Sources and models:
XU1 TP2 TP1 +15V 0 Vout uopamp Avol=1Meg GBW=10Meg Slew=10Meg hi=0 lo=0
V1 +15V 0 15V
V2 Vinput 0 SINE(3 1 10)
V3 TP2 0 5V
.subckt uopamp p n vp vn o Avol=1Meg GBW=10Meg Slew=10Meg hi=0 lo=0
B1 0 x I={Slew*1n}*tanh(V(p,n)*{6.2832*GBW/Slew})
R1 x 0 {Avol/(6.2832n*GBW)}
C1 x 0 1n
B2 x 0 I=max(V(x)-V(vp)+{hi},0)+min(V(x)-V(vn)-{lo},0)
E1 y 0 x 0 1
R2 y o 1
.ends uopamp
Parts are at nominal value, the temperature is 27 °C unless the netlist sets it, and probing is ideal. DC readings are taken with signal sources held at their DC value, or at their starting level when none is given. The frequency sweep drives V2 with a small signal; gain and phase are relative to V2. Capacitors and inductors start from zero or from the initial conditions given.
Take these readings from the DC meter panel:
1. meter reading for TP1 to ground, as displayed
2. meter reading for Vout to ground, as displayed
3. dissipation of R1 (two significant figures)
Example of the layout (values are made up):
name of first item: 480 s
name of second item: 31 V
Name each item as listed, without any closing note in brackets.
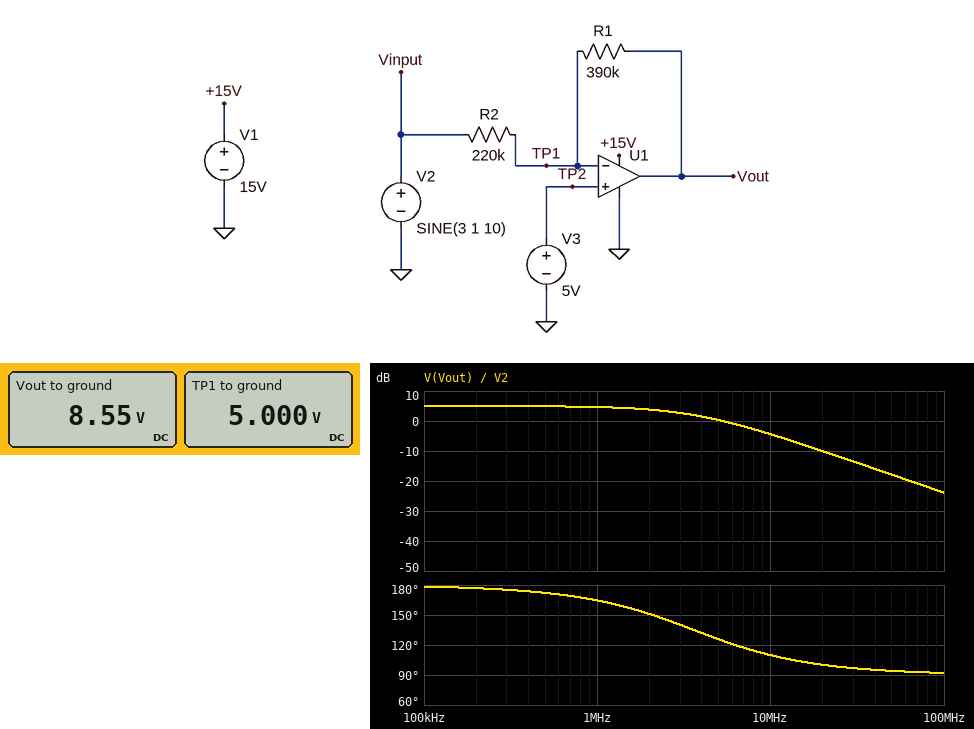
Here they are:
meter reading for TP1 to ground, as displayed: 5.000 V
meter reading for Vout to ground, as displayed: 8.55 V
dissipation of R1: 32 µW
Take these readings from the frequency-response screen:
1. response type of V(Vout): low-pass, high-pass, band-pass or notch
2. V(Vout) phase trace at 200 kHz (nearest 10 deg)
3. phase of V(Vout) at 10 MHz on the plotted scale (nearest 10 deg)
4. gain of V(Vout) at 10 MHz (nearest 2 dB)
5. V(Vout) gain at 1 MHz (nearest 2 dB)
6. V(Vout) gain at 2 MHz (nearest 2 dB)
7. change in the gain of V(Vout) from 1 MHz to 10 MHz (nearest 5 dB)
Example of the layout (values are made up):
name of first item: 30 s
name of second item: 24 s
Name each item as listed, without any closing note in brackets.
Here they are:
response type of V(Vout): low-pass, high-pass, band-pass or notch: low-pass
V(Vout) phase trace at 200 kHz: 180 deg
phase of V(Vout) at 10 MHz on the plotted scale: 110 deg
gain of V(Vout) at 10 MHz: -4 dB
V(Vout) gain at 1 MHz: 4 dB
V(Vout) gain at 2 MHz: 4 dB
change in the gain of V(Vout) from 1 MHz to 10 MHz: -10 dB
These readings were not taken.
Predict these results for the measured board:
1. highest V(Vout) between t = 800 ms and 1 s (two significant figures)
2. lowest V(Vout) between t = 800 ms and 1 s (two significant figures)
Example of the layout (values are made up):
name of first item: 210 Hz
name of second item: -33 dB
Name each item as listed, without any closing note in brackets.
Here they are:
highest V(Vout) between t = 800 ms and 1 s: 10 V
lowest V(Vout) between t = 800 ms and 1 s: 6.8 V
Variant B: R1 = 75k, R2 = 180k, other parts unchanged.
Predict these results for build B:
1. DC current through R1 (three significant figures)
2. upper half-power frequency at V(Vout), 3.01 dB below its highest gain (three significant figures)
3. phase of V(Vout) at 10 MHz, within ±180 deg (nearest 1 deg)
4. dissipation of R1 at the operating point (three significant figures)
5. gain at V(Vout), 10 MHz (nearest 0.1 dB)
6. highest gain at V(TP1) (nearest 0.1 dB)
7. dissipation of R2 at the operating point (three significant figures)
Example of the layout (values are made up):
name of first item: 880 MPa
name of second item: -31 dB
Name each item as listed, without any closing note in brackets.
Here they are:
DC current through R1: 11.1 µA
upper half-power frequency at V(Vout), 3.01 dB below its highest gain: 7.06 MHz
phase of V(Vout) at 10 MHz, within ±180 deg: 125 deg
dissipation of R1 at the operating point: 9.26 µW
gain at V(Vout), 10 MHz: -12.4 dB
highest gain at V(TP1): -10.6 dB
dissipation of R2 at the operating point: 22.2 µW
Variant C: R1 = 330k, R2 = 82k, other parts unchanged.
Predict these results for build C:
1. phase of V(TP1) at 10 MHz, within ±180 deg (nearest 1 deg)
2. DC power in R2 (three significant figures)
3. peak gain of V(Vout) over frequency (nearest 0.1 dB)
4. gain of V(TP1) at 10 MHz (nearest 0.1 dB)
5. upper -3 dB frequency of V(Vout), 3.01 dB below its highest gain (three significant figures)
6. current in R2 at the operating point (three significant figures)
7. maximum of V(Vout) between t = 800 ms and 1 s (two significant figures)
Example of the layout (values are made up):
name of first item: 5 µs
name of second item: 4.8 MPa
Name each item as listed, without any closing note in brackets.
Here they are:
phase of V(TP1) at 10 MHz, within ±180 deg: 11 deg
DC power in R2: 48.8 µW
peak gain of V(Vout) over frequency: 12.1 dB
gain of V(TP1) at 10 MHz: -2.1 dB
upper -3 dB frequency of V(Vout), 3.01 dB below its highest gain: 1.99 MHz
current in R2 at the operating point: 24.4 µA
maximum of V(Vout) between t = 800 ms and 1 s: 15 V
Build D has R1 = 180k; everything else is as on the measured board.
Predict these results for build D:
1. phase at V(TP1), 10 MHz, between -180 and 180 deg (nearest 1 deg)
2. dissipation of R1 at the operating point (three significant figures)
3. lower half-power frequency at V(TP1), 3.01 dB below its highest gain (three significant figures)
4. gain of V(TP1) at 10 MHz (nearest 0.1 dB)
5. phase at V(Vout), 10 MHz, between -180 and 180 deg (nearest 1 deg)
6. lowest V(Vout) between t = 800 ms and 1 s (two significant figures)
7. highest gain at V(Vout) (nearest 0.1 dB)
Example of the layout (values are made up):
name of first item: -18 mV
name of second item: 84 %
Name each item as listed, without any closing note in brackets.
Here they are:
phase at V(TP1), 10 MHz, between -180 and 180 deg: 29 deg
dissipation of R1 at the operating point: 14.9 µW
lower half-power frequency at V(TP1), 3.01 dB below its highest gain: 5.50 MHz
gain of V(TP1) at 10 MHz: -8.1 dB
phase at V(Vout), 10 MHz, between -180 and 180 deg: 119 deg
lowest V(Vout) between t = 800 ms and 1 s: 5.8 V
highest gain at V(Vout): -1.7 dB
